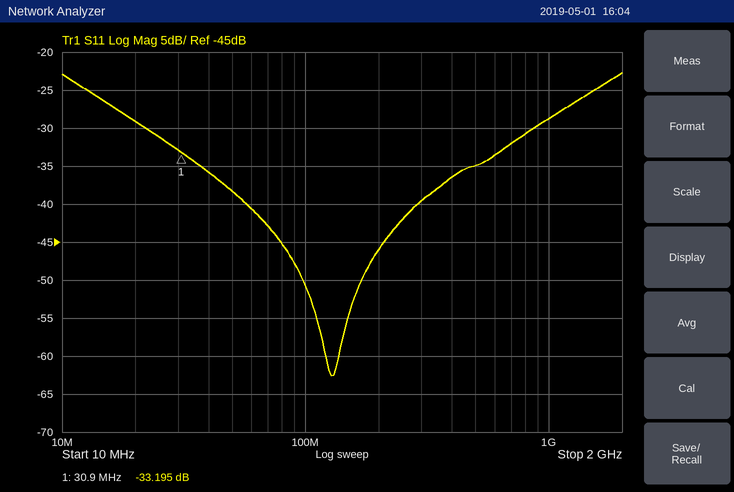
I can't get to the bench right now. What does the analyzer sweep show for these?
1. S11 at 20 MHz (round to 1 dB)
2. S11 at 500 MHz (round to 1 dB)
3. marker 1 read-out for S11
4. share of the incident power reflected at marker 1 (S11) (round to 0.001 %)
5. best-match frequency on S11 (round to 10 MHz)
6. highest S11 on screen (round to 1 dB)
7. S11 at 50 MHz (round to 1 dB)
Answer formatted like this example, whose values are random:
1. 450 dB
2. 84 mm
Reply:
1. -29 dB
2. -35 dB
3. -33.195 dB
4. 0.048 %
5. 130 MHz
6. -23 dB
7. -38 dB
